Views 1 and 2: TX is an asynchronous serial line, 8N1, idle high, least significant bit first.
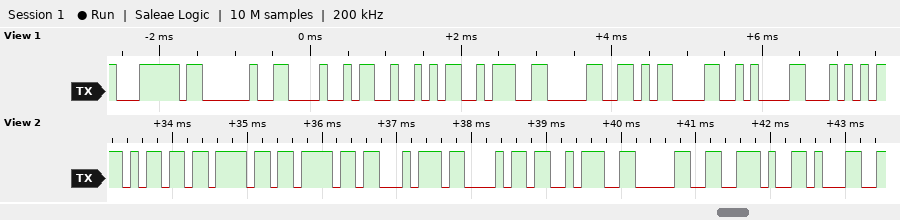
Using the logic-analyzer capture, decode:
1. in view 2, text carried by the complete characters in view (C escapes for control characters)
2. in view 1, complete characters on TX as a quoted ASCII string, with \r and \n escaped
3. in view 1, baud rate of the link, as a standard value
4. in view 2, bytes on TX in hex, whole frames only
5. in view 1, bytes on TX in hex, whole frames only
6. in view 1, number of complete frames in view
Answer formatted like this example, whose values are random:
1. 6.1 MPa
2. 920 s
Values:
1. "mooth:0.1"
2. "| HR:0\r\nT"
3. 9600 baud
4. 6D 6F 6F 74 68 3A 30 2E 31
5. 7C 20 48 52 3A 30 0D 0A 54
6. 9
